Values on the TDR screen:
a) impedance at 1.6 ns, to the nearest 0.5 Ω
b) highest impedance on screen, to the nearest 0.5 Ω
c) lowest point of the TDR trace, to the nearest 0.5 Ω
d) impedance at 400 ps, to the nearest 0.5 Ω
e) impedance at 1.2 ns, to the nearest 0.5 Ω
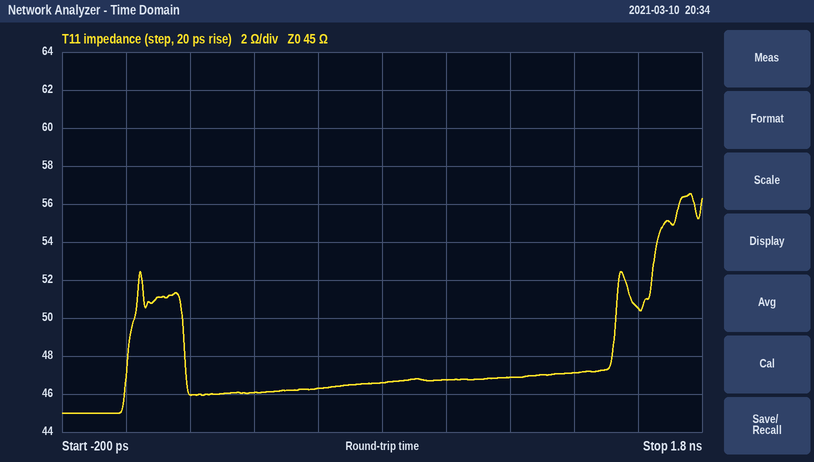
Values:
50.5 Ω
56.5 Ω
45.0 Ω
46.0 Ω
47.0 Ω
